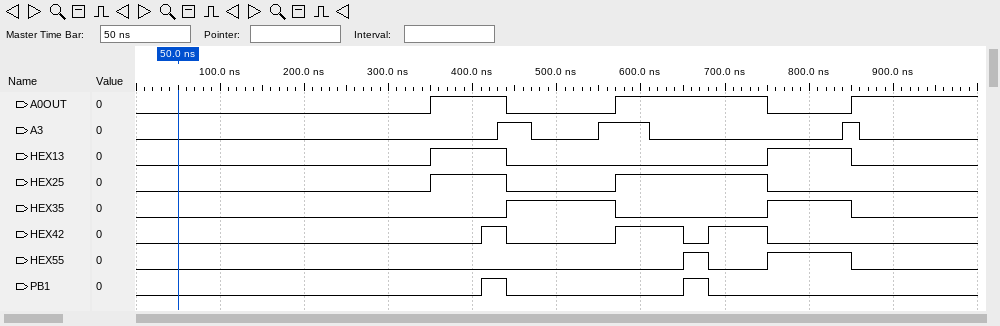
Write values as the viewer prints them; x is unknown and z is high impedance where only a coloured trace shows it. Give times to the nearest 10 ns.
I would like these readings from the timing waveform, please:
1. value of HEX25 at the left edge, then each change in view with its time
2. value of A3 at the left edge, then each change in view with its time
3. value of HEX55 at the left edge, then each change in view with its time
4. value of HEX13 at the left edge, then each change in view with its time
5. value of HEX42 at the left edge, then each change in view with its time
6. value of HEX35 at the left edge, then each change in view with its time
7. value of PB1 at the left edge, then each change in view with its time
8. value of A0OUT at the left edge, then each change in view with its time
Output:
0, 1 at 350 ns, 0 at 440 ns, 1 at 570 ns, 0 at 750 ns
0, 1 at 430 ns, 0 at 470 ns, 1 at 550 ns, 0 at 610 ns, 1 at 840 ns, 0 at 860 ns
0, 1 at 650 ns, 0 at 680 ns, 1 at 750 ns, 0 at 850 ns
0, 1 at 350 ns, 0 at 440 ns, 1 at 750 ns, 0 at 850 ns
0, 1 at 410 ns, 0 at 440 ns, 1 at 570 ns, 0 at 650 ns, 1 at 680 ns, 0 at 750 ns
0, 1 at 440 ns, 0 at 570 ns, 1 at 750 ns, 0 at 850 ns
0, 1 at 410 ns, 0 at 440 ns, 1 at 650 ns, 0 at 680 ns
0, 1 at 350 ns, 0 at 440 ns, 1 at 570 ns, 0 at 750 ns, 1 at 850 ns
